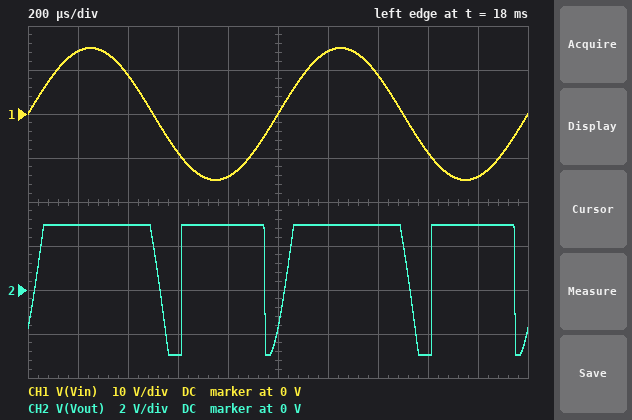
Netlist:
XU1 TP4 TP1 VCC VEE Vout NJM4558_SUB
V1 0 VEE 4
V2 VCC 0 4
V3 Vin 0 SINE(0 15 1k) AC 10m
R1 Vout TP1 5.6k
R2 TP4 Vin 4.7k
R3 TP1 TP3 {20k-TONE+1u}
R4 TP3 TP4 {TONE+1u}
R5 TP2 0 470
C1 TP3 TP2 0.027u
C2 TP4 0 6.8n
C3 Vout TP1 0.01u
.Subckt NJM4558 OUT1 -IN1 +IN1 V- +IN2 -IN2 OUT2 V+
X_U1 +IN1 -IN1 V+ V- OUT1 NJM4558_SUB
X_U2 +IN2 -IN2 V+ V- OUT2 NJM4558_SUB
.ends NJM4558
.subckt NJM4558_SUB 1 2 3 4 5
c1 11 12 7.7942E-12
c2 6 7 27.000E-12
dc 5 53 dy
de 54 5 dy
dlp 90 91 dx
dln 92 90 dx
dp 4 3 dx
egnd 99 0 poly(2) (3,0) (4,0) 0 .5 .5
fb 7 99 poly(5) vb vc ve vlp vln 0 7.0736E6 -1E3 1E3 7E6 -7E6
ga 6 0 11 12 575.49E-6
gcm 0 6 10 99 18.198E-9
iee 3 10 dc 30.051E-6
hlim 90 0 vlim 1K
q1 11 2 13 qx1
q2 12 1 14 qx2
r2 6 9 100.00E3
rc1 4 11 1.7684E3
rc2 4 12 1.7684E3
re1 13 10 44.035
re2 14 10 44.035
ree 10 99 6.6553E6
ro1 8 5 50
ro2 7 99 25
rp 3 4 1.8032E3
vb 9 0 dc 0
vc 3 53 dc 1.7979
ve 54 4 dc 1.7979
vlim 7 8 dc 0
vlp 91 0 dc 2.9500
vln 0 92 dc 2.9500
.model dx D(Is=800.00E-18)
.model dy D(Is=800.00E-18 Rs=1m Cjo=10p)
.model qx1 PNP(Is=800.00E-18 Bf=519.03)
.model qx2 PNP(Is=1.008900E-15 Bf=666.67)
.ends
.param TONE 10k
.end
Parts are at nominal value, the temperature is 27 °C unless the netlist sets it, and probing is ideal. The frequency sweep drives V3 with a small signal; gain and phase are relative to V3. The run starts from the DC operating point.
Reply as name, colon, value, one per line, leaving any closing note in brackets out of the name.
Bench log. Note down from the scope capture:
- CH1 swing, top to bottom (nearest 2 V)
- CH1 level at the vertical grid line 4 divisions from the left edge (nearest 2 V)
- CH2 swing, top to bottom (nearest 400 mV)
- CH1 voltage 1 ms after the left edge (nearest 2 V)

CH1 swing, top to bottom: 30 V
CH1 level at the vertical grid line 4 divisions from the left edge: -14 V
CH2 swing, top to bottom: 6.0 V
CH1 voltage 1 ms after the left edge: 0 V
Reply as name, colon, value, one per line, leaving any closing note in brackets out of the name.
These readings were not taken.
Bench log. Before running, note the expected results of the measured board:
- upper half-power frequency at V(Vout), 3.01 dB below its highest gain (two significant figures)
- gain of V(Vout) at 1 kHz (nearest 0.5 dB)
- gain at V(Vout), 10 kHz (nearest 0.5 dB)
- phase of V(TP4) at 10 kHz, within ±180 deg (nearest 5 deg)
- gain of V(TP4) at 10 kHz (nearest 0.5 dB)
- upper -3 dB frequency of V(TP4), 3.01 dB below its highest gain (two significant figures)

upper half-power frequency at V(Vout), 3.01 dB below its highest gain: 4.1 kHz
gain of V(Vout) at 1 kHz: 0 dB
gain at V(Vout), 10 kHz: -7.5 dB
phase of V(TP4) at 10 kHz, within ±180 deg: -55 deg
gain of V(TP4) at 10 kHz: -8.0 dB
upper -3 dB frequency of V(TP4), 3.01 dB below its highest gain: 1.7 kHz
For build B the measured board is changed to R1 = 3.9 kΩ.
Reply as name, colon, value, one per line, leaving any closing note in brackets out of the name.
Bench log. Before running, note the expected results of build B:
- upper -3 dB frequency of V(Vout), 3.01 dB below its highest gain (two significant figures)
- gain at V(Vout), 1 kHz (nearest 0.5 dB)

upper -3 dB frequency of V(Vout), 3.01 dB below its highest gain: 4.3 kHz
gain at V(Vout), 1 kHz: -0.5 dB
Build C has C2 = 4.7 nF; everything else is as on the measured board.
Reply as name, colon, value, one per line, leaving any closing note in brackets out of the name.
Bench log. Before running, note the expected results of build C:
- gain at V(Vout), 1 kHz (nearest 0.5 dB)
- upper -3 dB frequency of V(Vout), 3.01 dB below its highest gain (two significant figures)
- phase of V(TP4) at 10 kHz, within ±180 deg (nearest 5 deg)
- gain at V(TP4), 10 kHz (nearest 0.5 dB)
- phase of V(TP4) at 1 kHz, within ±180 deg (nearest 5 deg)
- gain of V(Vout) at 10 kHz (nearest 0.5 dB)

gain at V(Vout), 1 kHz: 0.5 dB
upper -3 dB frequency of V(Vout), 3.01 dB below its highest gain: 4.9 kHz
phase of V(TP4) at 10 kHz, within ±180 deg: -45 deg
gain at V(TP4), 10 kHz: -6.0 dB
phase of V(TP4) at 1 kHz, within ±180 deg: -15 deg
gain of V(Vout) at 10 kHz: -5.5 dB
